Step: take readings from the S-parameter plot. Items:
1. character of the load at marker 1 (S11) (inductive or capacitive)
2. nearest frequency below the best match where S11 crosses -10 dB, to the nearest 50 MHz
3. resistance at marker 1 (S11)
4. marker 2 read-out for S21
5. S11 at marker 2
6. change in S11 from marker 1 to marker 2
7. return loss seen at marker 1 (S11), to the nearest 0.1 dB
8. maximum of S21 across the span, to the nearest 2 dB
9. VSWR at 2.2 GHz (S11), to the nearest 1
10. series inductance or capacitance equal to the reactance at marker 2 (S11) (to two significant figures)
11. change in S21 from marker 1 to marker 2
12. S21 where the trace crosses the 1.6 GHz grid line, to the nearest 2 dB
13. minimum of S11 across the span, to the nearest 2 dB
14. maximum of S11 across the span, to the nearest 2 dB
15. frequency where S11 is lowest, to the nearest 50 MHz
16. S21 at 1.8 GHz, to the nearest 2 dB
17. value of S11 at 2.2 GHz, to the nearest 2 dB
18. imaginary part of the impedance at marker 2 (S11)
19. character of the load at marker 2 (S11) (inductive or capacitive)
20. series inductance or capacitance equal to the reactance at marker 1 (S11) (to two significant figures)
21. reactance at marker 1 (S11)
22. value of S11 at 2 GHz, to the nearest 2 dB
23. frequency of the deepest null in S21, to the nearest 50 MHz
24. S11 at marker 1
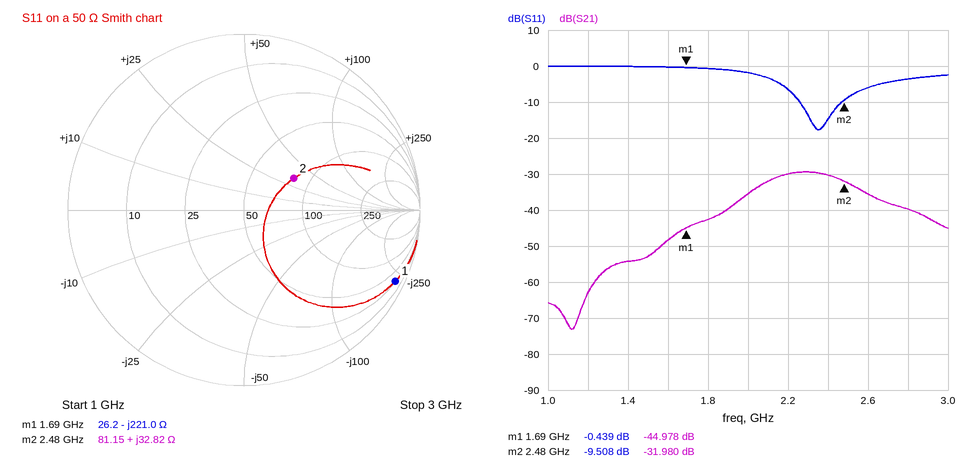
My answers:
capacitive
2.25 GHz
26.2 Ω
-31.980 dB
-9.508 dB
-9.069 dB
0.4 dB
-30 dB
3
2.1 nH
12.998 dB
-48 dB
-18 dB
0 dB
2.35 GHz
-42 dB
-6 dB
+32.82 Ω
inductive
430 fF
-221.0 Ω
-2 dB
1.10 GHz
-0.439 dB
